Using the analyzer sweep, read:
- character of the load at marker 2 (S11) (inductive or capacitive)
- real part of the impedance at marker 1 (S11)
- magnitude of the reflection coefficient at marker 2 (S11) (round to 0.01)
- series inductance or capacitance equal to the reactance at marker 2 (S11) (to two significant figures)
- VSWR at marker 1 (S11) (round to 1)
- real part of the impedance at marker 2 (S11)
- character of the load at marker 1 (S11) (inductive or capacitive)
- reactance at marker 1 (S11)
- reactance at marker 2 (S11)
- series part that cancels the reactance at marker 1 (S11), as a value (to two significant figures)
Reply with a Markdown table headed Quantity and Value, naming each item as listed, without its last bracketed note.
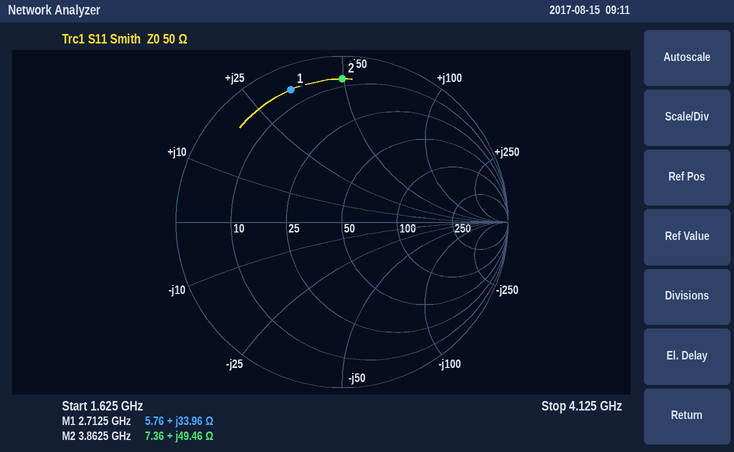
| Quantity | Value |
|---|---|
| character of the load at marker 2 (S11) | inductive |
| real part of the impedance at marker 1 | 5.76 Ω |
| magnitude of the reflection coefficient at marker 2 (S11) | 0.86 |
| series inductance or capacitance equal to the reactance at marker 2 (S11) | 2.0 nH |
| VSWR at marker 1 (S11) | 13 |
| real part of the impedance at marker 2 | 7.36 Ω |
| character of the load at marker 1 (S11) | inductive |
| reactance at marker 1 | +33.96 Ω |
| reactance at marker 2 | +49.46 Ω |
| series part that cancels the reactance at marker 1 (S11), as a value | 1.7 pF |
